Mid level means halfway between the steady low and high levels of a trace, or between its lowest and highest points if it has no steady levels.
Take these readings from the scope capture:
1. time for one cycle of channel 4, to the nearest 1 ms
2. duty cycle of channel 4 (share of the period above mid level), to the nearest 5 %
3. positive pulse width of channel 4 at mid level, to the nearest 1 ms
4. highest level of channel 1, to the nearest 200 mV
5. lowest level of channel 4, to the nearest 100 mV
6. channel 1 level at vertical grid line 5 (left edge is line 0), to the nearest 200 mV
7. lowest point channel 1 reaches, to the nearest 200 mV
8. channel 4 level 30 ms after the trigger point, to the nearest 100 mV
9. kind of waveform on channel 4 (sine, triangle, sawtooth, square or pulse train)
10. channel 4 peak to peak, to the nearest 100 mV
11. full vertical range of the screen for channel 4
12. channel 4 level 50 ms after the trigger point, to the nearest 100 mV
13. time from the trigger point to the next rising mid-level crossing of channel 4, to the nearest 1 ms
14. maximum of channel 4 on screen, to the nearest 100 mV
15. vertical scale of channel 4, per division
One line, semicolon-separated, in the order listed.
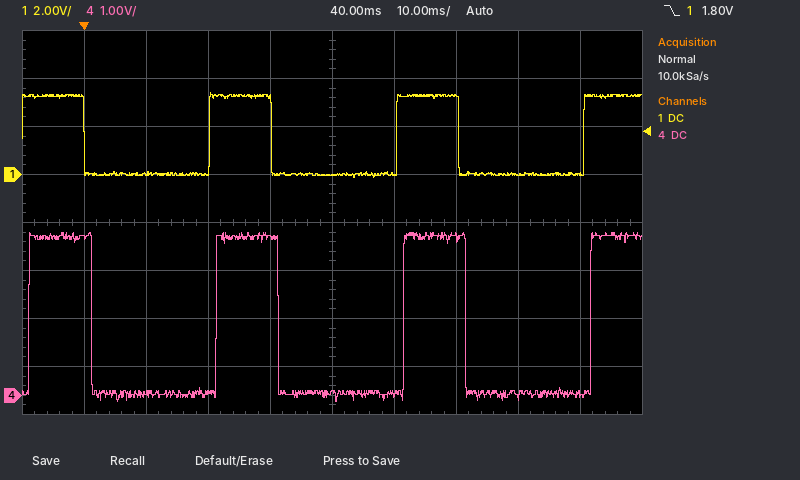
30 ms; 35 %; 10 ms; 3.4 V; -100 mV; 0.0 V; -200 mV; 3.3 V; pulse train; 3.5 V; 8 V; 0.0 V; 21 ms; 3.4 V; 1 V
